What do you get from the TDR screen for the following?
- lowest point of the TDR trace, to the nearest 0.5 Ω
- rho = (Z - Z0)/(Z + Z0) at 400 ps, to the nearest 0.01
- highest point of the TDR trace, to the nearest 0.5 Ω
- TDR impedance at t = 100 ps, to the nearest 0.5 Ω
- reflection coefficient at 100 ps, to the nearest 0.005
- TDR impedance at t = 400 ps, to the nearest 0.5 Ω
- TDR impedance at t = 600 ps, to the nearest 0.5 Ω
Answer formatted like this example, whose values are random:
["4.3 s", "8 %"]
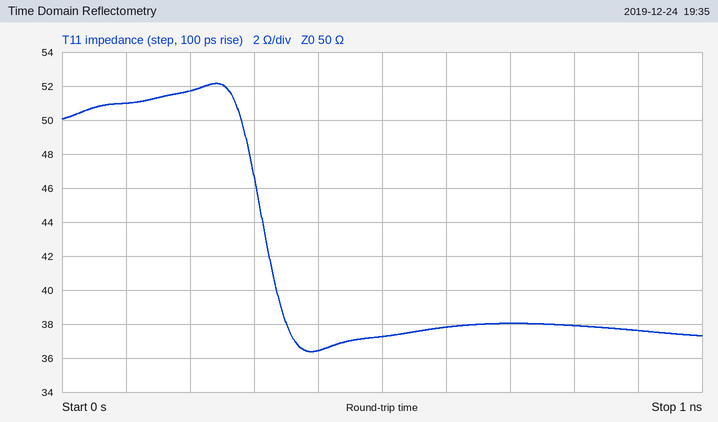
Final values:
["36.5 Ω", "-0.16", "52.0 Ω", "51.0 Ω", "+0.010", "36.5 Ω", "38.0 Ω"]
